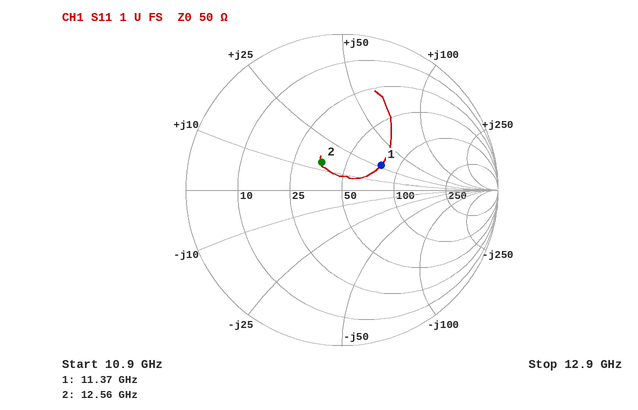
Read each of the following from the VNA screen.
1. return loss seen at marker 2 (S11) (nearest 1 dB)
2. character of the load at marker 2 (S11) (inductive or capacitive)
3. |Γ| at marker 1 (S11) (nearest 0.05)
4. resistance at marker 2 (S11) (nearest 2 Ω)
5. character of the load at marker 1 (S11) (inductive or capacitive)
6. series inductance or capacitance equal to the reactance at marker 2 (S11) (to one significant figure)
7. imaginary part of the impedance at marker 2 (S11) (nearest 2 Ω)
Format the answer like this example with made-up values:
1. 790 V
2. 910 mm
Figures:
1. 13 dB
2. inductive
3. 0.30
4. 36 Ω
5. inductive
6. 200 pH
7. +14 Ω
